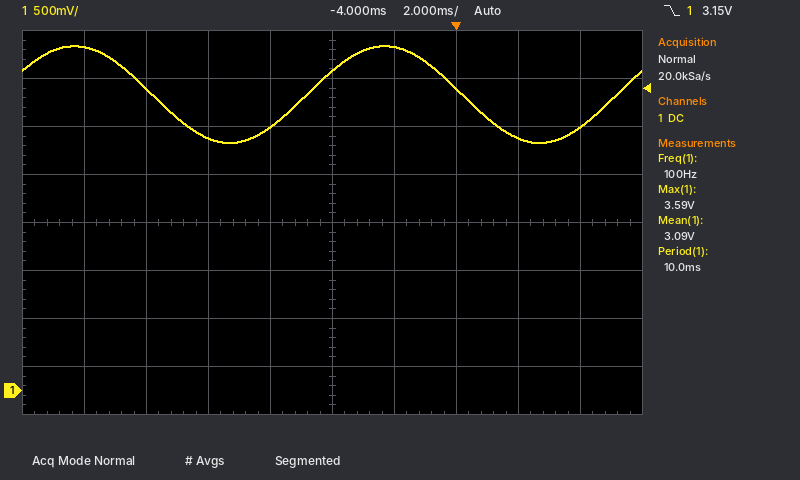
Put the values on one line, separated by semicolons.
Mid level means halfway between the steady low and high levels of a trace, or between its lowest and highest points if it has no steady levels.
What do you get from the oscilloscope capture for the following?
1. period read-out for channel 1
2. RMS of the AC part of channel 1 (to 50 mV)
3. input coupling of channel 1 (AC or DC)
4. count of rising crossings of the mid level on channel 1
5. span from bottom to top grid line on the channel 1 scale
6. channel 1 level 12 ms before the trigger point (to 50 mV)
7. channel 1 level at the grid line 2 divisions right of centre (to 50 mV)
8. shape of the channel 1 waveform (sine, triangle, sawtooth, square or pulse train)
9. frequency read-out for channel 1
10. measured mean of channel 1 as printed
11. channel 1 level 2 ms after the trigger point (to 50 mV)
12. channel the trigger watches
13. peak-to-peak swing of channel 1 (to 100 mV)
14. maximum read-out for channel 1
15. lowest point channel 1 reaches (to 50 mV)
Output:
10.0 ms; 350 mV; DC; 2; 4 V; 3.60 V; 3.15 V; sine; 100 Hz; 3.09 V; 2.65 V; channel 1; 1.00 V; 3.59 V; 2.60 V
